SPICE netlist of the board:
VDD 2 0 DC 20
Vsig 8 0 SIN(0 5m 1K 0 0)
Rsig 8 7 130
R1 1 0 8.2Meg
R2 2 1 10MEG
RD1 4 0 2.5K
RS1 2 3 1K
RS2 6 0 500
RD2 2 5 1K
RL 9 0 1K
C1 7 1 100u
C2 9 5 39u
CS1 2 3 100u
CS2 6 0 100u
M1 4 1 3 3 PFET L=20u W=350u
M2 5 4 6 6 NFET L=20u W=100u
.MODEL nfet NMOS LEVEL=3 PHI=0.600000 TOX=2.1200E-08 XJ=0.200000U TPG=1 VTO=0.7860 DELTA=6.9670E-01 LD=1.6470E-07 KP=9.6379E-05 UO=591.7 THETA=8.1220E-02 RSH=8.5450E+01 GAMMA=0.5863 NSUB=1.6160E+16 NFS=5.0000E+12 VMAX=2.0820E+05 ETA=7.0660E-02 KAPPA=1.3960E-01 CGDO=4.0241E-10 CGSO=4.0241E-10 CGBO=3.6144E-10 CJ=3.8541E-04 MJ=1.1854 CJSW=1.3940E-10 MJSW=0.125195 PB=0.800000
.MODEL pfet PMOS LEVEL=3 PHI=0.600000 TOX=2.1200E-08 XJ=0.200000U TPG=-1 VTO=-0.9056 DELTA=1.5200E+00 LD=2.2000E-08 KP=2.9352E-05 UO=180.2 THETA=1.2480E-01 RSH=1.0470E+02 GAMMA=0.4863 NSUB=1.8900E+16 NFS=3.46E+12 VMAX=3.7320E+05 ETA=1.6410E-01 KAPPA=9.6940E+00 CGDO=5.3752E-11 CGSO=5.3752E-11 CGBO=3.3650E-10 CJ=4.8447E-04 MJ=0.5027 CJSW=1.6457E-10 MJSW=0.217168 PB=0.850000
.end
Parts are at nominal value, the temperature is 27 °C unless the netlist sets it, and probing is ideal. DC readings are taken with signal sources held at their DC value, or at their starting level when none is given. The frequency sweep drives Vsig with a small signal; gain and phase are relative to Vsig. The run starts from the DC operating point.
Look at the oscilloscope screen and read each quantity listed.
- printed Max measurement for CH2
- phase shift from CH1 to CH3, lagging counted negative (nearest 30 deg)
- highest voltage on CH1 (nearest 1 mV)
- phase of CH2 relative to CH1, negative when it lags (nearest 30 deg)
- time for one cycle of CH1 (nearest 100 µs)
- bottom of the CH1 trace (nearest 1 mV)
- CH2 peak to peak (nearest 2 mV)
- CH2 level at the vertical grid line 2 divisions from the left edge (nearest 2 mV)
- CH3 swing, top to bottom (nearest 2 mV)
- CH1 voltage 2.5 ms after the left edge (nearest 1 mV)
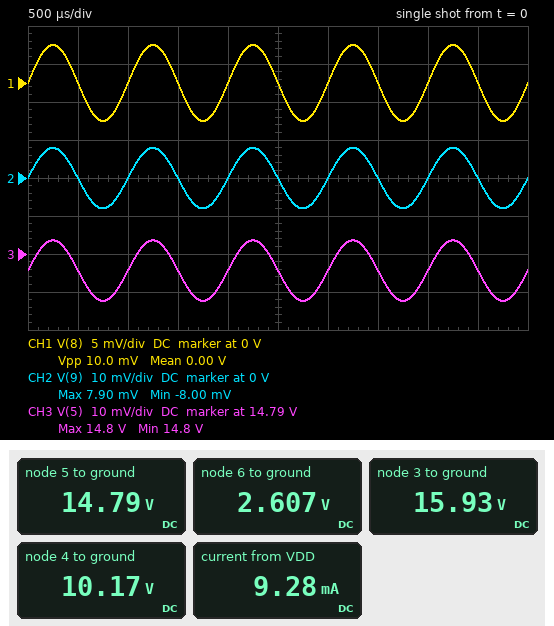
7.90 mV
0 deg
5 mV
0 deg
1.0 ms
-5 mV
16 mV
0 V
16 mV
0 V
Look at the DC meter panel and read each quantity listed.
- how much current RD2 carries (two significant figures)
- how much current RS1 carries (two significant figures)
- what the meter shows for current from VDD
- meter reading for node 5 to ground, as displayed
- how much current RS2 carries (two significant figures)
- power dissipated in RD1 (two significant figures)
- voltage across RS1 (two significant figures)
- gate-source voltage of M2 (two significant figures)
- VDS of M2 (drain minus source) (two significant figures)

5.2 mA
4.1 mA
9.28 mA
14.79 V
5.2 mA
41 mW
4.1 V
7.6 V
12 V
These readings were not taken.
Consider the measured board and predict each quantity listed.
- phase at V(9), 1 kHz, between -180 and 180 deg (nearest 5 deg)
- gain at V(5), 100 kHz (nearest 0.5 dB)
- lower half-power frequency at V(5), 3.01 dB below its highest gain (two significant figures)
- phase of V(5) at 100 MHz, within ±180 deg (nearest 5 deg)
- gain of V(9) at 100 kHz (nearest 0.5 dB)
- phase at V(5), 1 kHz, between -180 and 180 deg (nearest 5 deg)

0 deg
4.0 dB
1.7 Hz
-125 deg
4.0 dB
0 deg
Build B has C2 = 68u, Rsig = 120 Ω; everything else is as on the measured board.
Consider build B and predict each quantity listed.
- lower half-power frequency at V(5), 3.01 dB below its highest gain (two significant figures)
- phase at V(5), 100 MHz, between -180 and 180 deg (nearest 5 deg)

3.6 Hz
-120 deg
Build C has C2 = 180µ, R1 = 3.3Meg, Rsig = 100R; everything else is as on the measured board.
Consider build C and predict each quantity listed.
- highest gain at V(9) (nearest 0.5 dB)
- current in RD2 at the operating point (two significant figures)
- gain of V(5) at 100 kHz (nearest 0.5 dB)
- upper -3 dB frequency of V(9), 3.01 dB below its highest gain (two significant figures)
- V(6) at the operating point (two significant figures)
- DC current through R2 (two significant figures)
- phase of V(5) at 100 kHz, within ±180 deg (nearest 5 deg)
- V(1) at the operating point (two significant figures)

-8.5 dB
6.4 mA
-18.5 dB
240 MHz
3.2 V
1.5 µA
0 deg
5.0 V
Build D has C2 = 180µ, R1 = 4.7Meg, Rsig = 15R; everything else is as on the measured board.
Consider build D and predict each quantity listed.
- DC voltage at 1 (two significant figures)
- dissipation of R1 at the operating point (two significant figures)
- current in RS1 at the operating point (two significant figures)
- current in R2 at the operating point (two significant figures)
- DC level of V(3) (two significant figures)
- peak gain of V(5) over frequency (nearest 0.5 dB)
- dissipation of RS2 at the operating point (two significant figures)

6.4 V
8.7 µW
4.6 mA
1.4 µA
15 V
-7.0 dB
19 mW
